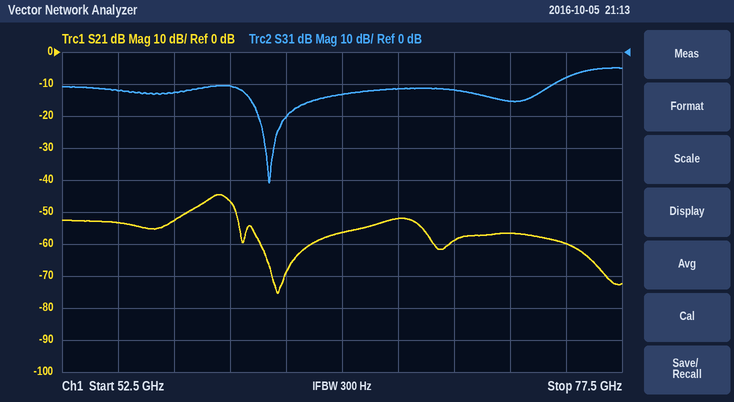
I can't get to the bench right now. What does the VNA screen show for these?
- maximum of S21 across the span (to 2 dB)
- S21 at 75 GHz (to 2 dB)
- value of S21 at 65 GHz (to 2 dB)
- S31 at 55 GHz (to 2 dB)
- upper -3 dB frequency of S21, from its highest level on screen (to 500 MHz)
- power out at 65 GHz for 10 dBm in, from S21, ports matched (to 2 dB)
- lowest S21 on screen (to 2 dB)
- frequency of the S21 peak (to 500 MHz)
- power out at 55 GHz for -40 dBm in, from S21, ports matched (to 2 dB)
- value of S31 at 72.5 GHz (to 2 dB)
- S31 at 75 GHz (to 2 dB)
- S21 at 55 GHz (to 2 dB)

-44 dB
-60 dB
-56 dB
-12 dB
60.0 GHz
-46 dBm
-76 dB
59.5 GHz
-94 dBm
-16 dB
-8 dB
-54 dB
